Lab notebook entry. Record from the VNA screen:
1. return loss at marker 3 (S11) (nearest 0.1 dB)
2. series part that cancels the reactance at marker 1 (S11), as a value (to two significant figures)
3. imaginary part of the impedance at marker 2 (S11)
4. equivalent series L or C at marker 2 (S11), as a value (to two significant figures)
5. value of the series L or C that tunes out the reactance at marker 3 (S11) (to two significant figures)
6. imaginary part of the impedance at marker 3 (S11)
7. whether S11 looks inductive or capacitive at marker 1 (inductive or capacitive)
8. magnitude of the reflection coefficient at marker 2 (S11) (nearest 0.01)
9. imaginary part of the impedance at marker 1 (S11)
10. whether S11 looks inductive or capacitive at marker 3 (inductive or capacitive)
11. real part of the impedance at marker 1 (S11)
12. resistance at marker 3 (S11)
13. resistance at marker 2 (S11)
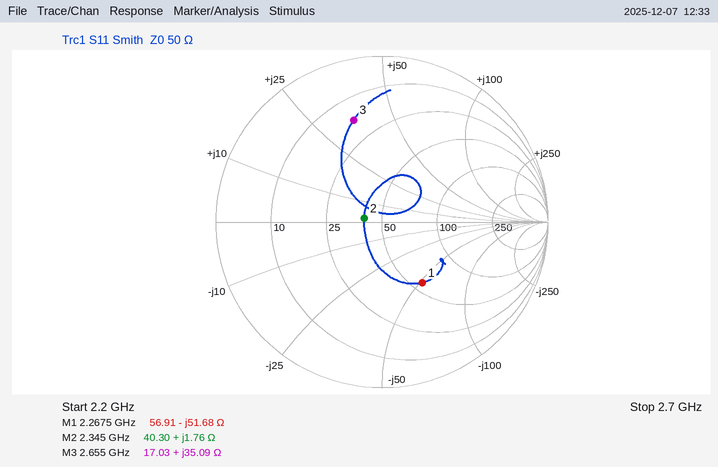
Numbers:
3.9 dB
3.6 nH
+1.76 Ω
120 pH
1.7 pF
+35.09 Ω
capacitive
0.11
-51.68 Ω
inductive
56.91 Ω
17.03 Ω
40.30 Ω
